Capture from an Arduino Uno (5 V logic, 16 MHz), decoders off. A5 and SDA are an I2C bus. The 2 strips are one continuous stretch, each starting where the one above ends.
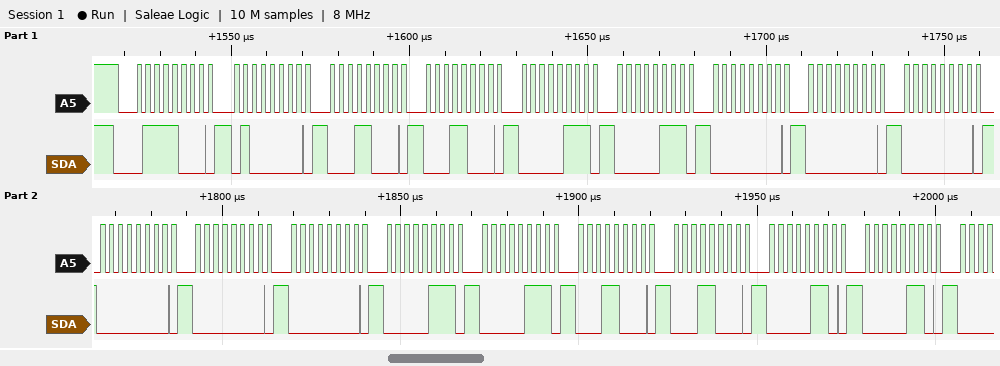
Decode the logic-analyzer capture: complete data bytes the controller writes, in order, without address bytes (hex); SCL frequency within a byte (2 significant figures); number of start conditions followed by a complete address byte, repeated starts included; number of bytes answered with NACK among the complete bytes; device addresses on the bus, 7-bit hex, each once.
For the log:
40 18 18 07 07 00 00 00 00 00 00 07 07 18 18 06 06
400 kHz
1
0
0x3C
